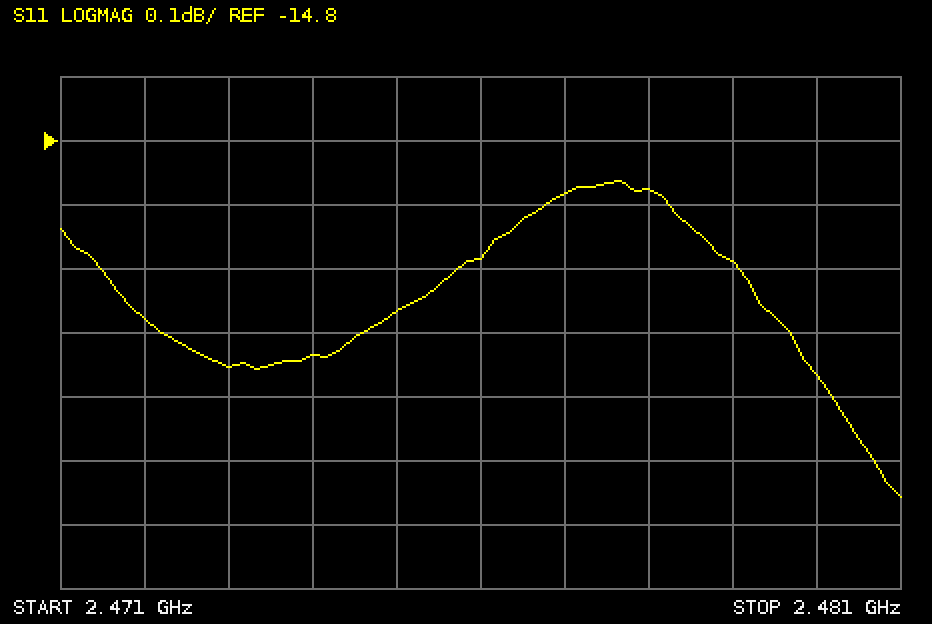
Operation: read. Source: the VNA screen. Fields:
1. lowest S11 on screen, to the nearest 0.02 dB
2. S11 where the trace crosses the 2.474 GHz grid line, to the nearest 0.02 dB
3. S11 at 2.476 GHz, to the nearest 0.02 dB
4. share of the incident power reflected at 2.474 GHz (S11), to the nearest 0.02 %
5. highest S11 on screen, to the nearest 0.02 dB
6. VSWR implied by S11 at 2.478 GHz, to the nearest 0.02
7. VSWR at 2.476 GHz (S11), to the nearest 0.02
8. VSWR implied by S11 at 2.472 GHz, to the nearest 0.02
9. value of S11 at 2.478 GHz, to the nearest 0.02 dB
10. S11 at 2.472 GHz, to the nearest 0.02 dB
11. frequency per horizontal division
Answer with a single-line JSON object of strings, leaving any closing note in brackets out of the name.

{"lowest S11 on screen, to the nearest 0.02 dB": "-15.36 dB", "S11 where the trace crosses the 2.474 GHz grid line, to the nearest 0.02 dB": "-15.14 dB", "S11 at 2.476 GHz, to the nearest 0.02 dB": "-14.98 dB", "share of the incident power reflected at 2.474 GHz (S11), to the nearest 0.02 %": "3.06 %", "highest S11 on screen, to the nearest 0.02 dB": "-14.86 dB", "VSWR implied by S11 at 2.478 GHz, to the nearest 0.02": "1.44", "VSWR at 2.476 GHz (S11), to the nearest 0.02": "1.44", "VSWR implied by S11 at 2.472 GHz, to the nearest 0.02": "1.42", "value of S11 at 2.478 GHz, to the nearest 0.02 dB": "-14.88 dB", "S11 at 2.472 GHz, to the nearest 0.02 dB": "-15.08 dB", "frequency per horizontal division": "1 MHz"}
